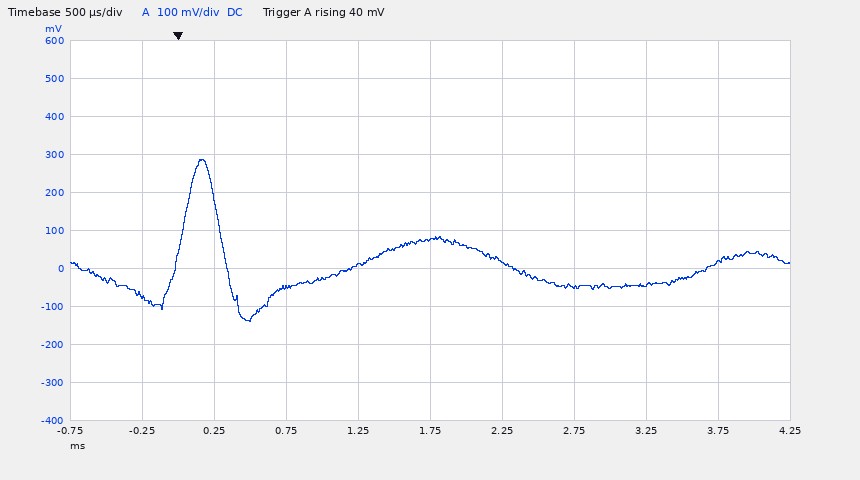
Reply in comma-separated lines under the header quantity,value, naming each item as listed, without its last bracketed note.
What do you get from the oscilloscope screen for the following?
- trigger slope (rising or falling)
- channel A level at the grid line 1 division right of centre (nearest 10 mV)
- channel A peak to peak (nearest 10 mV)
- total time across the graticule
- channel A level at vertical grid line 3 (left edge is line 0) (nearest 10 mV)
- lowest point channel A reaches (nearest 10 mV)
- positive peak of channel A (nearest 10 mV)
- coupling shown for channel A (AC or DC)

quantity,value
trigger slope,rising
channel A level at the grid line 1 division right of centre,20 mV
channel A peak to peak,430 mV
total time across the graticule,5 ms
channel A level at vertical grid line 3 (left edge is line 0),-50 mV
lowest point channel A reaches,-140 mV
positive peak of channel A,290 mV
coupling shown for channel A,DC
